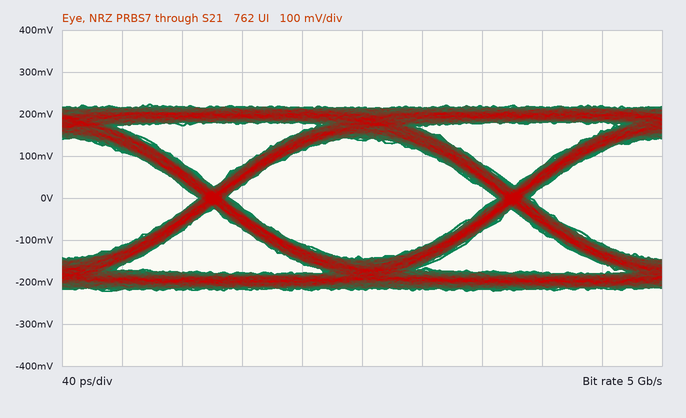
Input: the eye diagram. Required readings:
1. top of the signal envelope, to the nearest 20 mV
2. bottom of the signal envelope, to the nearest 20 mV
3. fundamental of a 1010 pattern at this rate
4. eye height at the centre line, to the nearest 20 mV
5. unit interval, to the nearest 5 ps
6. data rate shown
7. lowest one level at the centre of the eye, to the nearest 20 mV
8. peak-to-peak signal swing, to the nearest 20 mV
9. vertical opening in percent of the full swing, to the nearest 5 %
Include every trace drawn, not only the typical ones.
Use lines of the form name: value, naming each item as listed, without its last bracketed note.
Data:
top of the signal envelope, to the nearest 20 mV: 220 mV
bottom of the signal envelope, to the nearest 20 mV: -220 mV
fundamental of a 1010 pattern at this rate: 2.5 GHz
eye height at the centre line, to the nearest 20 mV: 280 mV
unit interval, to the nearest 5 ps: 200 ps
data rate shown: 5 Gb/s
lowest one level at the centre of the eye, to the nearest 20 mV: 140 mV
peak-to-peak signal swing, to the nearest 20 mV: 440 mV
vertical opening in percent of the full swing, to the nearest 5 %: 65 %
